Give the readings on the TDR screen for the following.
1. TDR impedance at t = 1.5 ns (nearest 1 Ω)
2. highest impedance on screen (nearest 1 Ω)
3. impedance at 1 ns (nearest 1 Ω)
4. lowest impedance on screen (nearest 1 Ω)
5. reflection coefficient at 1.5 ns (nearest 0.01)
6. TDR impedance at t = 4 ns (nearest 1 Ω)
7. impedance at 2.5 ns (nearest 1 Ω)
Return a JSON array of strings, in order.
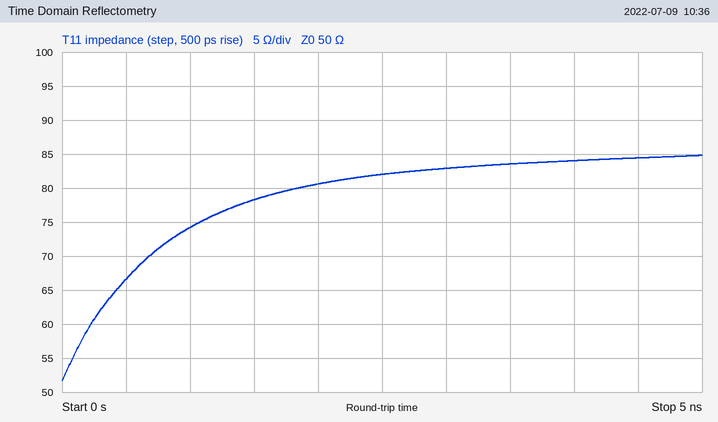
["78 Ω", "85 Ω", "74 Ω", "52 Ω", "+0.22", "84 Ω", "82 Ω"]
